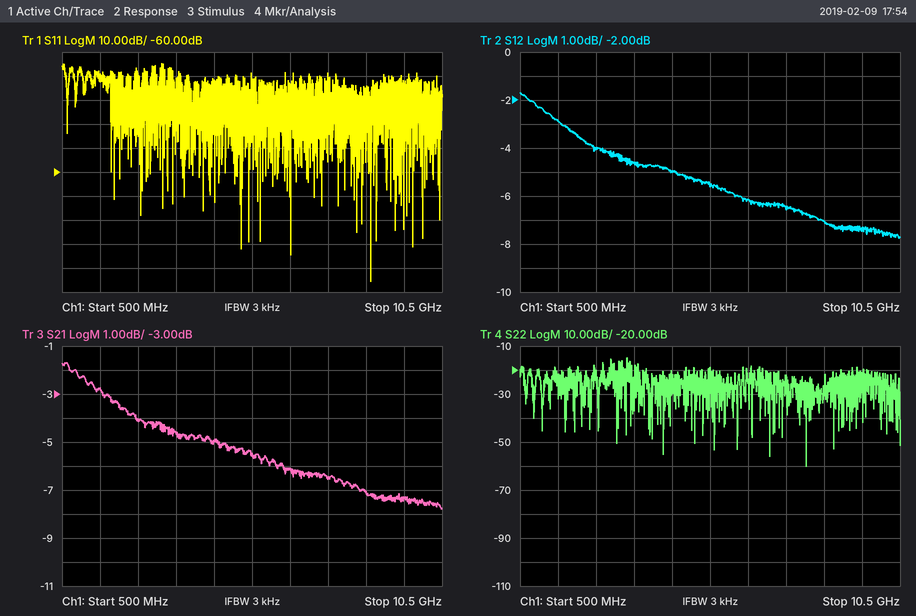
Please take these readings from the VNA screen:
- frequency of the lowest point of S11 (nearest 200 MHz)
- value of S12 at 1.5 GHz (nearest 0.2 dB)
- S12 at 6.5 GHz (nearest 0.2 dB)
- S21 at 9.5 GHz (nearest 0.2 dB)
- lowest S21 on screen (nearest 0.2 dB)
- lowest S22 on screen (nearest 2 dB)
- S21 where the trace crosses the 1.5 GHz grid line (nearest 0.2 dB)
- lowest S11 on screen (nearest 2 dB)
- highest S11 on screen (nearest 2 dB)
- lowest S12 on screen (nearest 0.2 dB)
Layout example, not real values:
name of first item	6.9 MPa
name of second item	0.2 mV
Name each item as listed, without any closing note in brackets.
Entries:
frequency of the lowest point of S11	8.6 GHz
value of S12 at 1.5 GHz	-2.8 dB
S12 at 6.5 GHz	-6.2 dB
S21 at 9.5 GHz	-7.4 dB
lowest S21 on screen	-7.8 dB
lowest S22 on screen	-60 dB
S21 where the trace crosses the 1.5 GHz grid line	-2.8 dB
lowest S11 on screen	-106 dB
highest S11 on screen	-14 dB
lowest S12 on screen	-7.8 dB
